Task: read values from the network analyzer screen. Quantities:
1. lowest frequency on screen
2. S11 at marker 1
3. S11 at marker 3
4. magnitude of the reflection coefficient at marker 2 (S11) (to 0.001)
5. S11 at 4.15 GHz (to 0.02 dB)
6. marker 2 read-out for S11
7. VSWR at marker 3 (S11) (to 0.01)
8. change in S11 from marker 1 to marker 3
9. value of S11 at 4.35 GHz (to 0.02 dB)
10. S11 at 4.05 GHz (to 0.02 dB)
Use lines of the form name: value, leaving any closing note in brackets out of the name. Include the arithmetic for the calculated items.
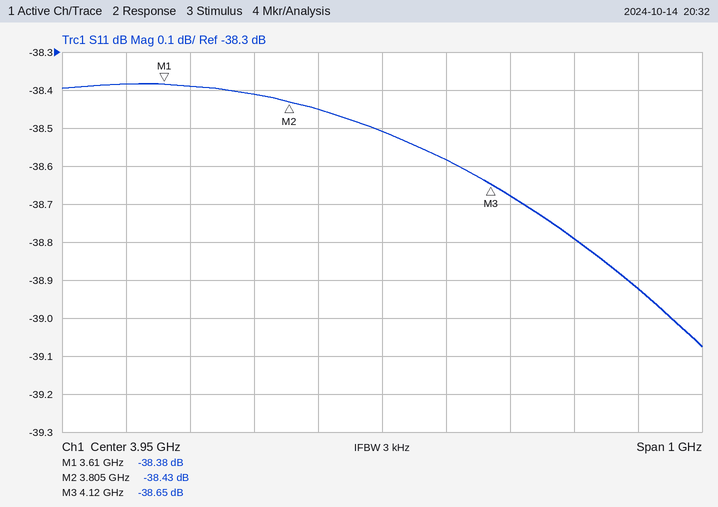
lowest frequency on screen: 3.45 GHz
S11 at marker 1: -38.38 dB
S11 at marker 3: -38.65 dB
magnitude of the reflection coefficient at marker 2 (S11): 10^(-38.43/20) ≈ 0.012
S11 at 4.15 GHz: -38.68 dB
marker 2 read-out for S11: -38.43 dB
VSWR at marker 3 (S11): (1 + 0.0117)/(1 − 0.0117) ≈ 1.02
change in S11 from marker 1 to marker 3: -38.65 − (-38.38) = -0.27 dB
value of S11 at 4.35 GHz: -38.92 dB
S11 at 4.05 GHz: -38.58 dB
